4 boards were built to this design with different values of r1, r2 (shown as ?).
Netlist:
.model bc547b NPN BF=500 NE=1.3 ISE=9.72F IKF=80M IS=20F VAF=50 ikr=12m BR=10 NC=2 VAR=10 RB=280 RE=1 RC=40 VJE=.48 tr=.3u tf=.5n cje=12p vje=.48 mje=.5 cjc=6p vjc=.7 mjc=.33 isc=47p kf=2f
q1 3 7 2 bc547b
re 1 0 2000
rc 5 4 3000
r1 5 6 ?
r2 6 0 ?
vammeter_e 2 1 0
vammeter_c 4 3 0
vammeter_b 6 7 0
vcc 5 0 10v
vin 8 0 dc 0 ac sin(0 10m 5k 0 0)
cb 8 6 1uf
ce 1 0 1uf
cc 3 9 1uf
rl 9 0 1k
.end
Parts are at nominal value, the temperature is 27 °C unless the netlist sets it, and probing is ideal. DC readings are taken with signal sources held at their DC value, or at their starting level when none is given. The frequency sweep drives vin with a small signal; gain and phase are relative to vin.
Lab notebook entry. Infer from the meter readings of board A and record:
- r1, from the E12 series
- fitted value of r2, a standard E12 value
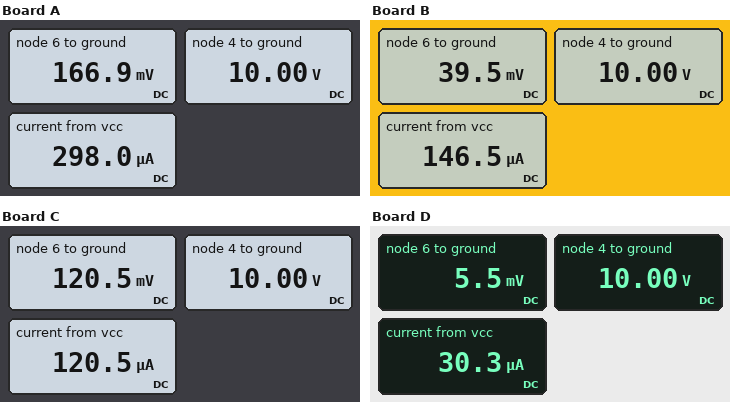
33 kΩ
560 Ω
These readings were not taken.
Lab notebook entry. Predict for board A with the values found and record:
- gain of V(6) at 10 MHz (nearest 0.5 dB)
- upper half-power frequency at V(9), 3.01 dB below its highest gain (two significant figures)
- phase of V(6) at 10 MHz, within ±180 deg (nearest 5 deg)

0 dB
150 MHz
0 deg
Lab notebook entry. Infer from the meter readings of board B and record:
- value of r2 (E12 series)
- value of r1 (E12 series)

270 Ω
68 kΩ
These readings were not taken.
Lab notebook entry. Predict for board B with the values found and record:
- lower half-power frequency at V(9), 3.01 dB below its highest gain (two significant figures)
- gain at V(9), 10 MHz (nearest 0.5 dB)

22 MHz
-19.0 dB
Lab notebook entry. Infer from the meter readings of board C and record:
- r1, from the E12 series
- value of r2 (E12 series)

82 kΩ
1 kΩ
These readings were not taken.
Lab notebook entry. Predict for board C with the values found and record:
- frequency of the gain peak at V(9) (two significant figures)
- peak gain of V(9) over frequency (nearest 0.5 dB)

58 MHz
-11.0 dB
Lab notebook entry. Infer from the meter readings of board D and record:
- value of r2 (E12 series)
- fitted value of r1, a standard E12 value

180 Ω
330 kΩ
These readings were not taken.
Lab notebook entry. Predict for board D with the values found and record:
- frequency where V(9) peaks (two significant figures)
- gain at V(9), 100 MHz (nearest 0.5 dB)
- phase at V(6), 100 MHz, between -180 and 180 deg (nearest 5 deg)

62 MHz
-11.0 dB
0 deg
